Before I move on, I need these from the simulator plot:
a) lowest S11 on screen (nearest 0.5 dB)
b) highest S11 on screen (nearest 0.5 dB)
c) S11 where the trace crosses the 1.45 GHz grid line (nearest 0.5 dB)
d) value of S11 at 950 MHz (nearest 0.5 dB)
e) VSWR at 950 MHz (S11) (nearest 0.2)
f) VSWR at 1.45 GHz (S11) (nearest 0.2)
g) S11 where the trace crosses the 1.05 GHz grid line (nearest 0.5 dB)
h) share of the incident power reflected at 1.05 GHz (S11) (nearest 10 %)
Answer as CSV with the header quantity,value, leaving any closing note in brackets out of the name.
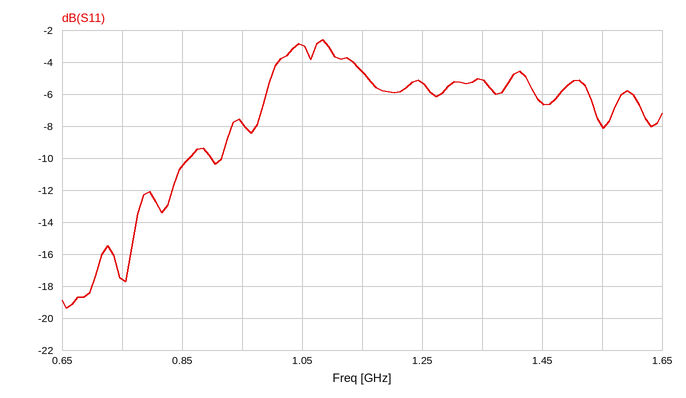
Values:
quantity,value
lowest S11 on screen,-19.5 dB
highest S11 on screen,-2.5 dB
S11 where the trace crosses the 1.45 GHz grid line,-6.5 dB
value of S11 at 950 MHz,-8.0 dB
VSWR at 950 MHz (S11),2.4
VSWR at 1.45 GHz (S11),2.8
S11 where the trace crosses the 1.05 GHz grid line,-3.0 dB
share of the incident power reflected at 1.05 GHz (S11),50 %
